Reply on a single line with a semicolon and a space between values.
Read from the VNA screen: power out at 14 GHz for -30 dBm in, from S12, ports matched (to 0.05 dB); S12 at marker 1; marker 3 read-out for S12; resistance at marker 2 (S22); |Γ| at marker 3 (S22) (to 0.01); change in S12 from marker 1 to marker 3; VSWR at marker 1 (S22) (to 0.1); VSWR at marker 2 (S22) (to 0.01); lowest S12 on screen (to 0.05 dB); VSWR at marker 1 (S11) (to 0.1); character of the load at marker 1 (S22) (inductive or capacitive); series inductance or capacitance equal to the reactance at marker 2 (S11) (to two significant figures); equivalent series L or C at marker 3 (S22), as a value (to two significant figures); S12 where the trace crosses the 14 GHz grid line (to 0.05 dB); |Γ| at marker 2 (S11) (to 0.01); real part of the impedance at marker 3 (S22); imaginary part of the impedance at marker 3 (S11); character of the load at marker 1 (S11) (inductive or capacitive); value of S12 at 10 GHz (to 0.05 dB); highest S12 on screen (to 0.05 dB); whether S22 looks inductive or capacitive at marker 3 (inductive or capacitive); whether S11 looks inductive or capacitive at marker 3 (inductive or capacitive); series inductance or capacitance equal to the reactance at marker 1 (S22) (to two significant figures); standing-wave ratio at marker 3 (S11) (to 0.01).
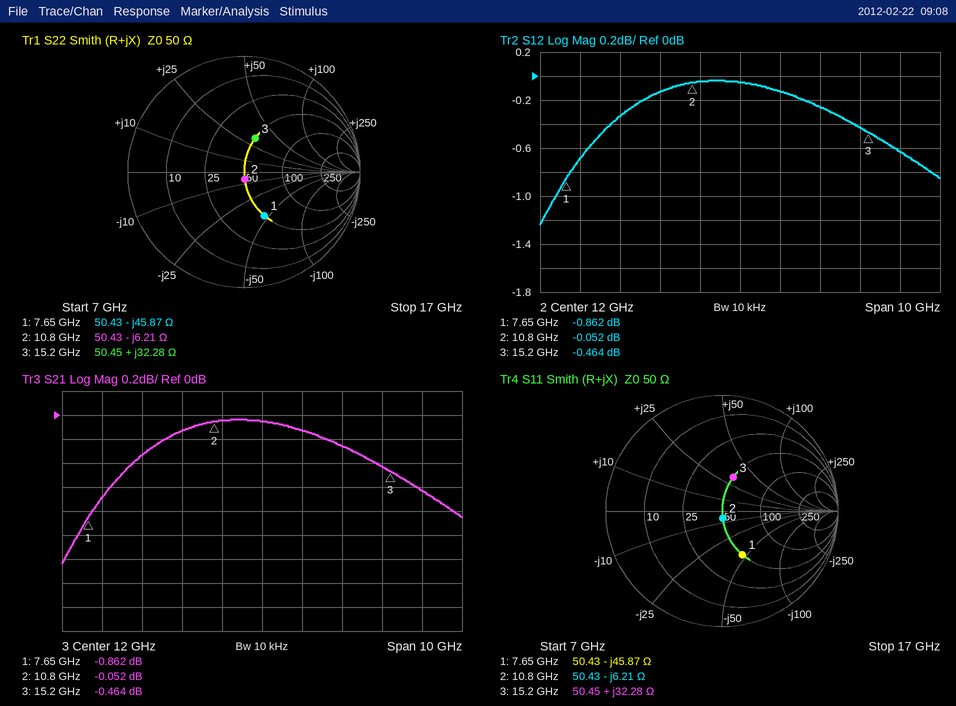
-30.25 dBm; -0.862 dB; -0.464 dB; 50.43 Ω; 0.31; 0.398 dB; 2.4; 1.13; -1.25 dB; 2.4; capacitive; 2.4 pF; 340 pH; -0.25 dB; 0.06; 50.45 Ω; +32.28 Ω; capacitive; -0.15 dB; -0.05 dB; inductive; inductive; 450 fF; 1.88
